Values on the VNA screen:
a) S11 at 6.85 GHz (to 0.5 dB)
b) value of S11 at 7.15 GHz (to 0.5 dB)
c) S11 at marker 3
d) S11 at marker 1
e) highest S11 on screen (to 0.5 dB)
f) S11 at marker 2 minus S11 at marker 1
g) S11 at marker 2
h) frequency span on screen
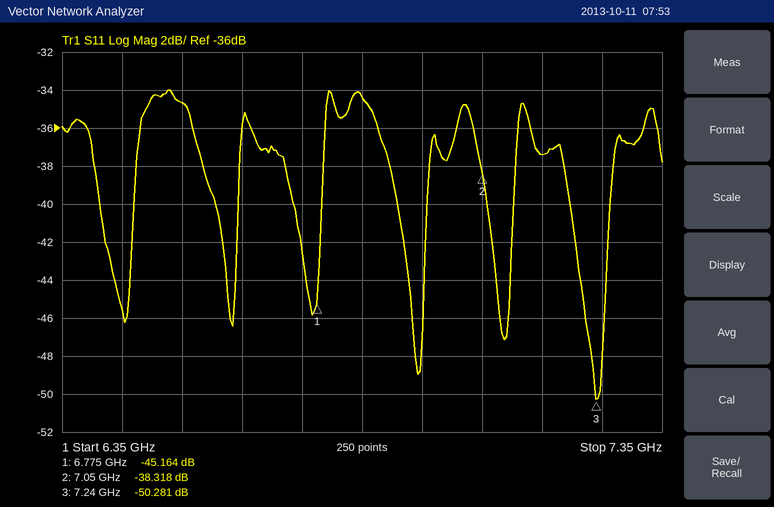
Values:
-34.5 dB
-37.5 dB
-50.281 dB
-45.164 dB
-34.0 dB
6.846 dB
-38.318 dB
1 GHz
